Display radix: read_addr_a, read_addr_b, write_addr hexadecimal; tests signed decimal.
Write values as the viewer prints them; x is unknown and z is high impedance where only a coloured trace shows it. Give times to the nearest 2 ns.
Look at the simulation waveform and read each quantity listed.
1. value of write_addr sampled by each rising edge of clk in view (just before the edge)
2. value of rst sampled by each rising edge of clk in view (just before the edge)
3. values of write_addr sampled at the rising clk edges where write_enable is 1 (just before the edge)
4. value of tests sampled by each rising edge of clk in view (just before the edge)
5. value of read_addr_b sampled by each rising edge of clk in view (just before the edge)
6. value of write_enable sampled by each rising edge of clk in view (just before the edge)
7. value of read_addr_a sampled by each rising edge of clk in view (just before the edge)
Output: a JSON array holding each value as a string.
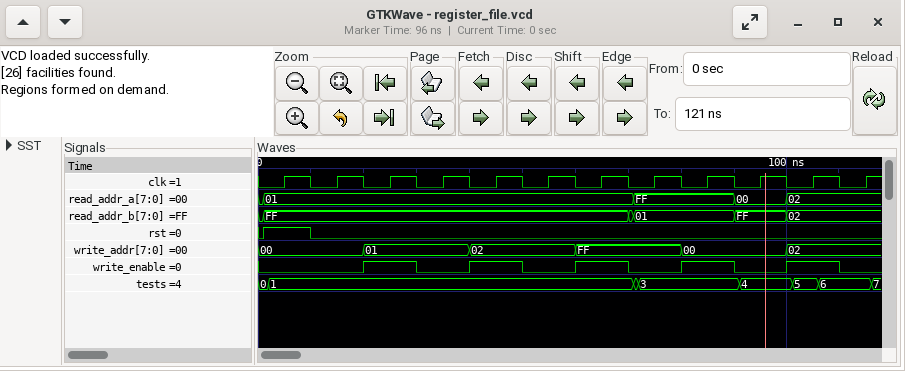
["00, 00, 01, 01, 02, 02, FF, FF, 00, 00, 02, 02", "1 0 0 0 0 0 0 0 0 0 0 0", "01, 02, FF, 00, 02", "1, 1, 1, 1, 1, 1, 1, 3, 3, 4, 5, 6", "FF, FF, FF, FF, FF, FF, FF, 01, 01, FF, 02, 02", "0 0 1 0 1 0 1 0 1 0 1 0", "01, 01, 01, 01, 01, 01, 01, FF, FF, 00, 02, 02"]
